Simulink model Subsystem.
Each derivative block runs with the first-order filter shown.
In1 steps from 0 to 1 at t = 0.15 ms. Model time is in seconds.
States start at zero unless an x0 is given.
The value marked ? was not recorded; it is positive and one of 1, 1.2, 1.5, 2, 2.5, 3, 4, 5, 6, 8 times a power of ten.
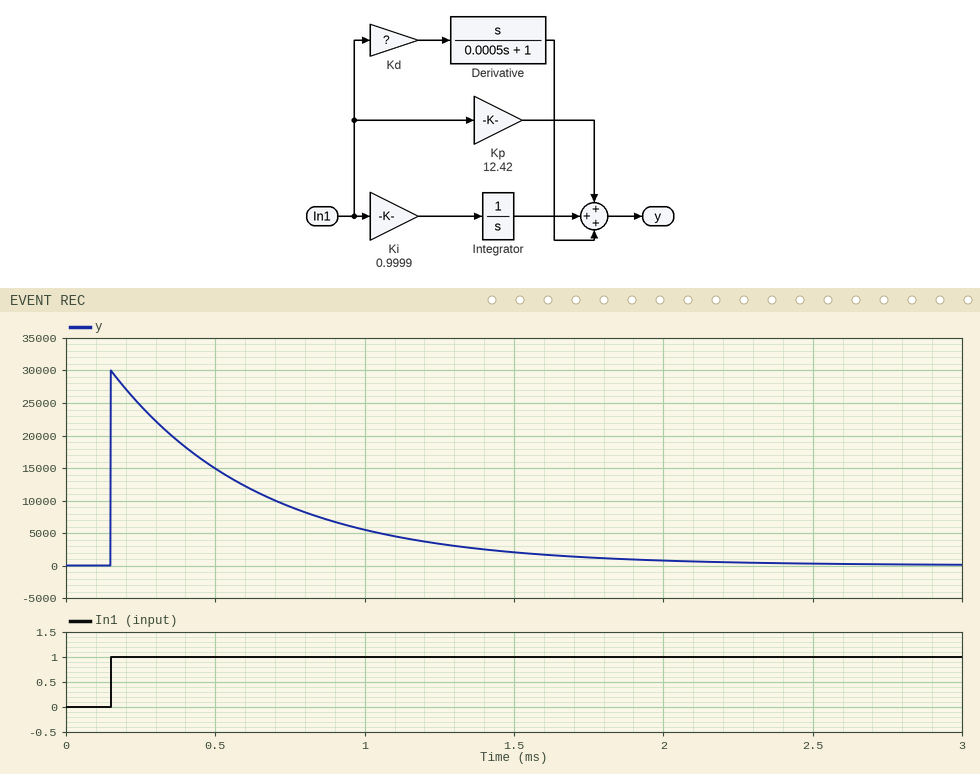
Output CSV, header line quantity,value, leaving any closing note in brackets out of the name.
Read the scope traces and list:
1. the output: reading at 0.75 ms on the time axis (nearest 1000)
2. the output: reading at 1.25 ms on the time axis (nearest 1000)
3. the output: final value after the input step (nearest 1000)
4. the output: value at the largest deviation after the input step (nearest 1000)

quantity,value
the output: reading at 0.75 ms on the time axis,9000
the output: reading at 1.25 ms on the time axis,3000
the output: final value after the input step,0
the output: value at the largest deviation after the input step,30000
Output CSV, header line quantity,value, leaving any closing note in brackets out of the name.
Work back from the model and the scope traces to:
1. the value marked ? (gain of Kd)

quantity,value
the value marked ?,15
